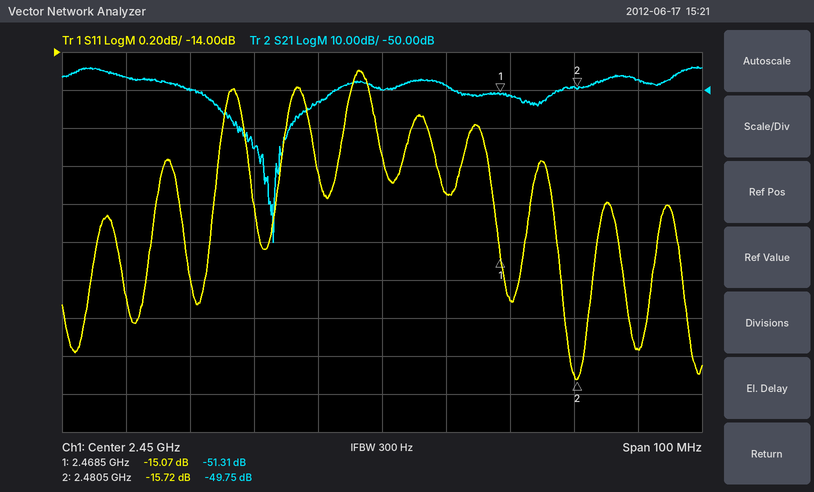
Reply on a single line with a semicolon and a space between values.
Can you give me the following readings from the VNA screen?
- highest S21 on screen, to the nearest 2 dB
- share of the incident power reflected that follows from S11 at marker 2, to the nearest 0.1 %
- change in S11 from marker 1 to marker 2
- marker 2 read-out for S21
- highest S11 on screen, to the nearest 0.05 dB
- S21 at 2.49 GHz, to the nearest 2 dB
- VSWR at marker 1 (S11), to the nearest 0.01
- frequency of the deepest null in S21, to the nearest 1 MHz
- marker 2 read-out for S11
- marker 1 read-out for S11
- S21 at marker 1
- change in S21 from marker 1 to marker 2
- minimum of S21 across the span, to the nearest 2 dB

-44 dB; 2.7 %; -0.65 dB; -49.75 dB; -14.10 dB; -48 dB; 1.43; 2.433 GHz; -15.72 dB; -15.07 dB; -51.31 dB; 1.56 dB; -90 dB
